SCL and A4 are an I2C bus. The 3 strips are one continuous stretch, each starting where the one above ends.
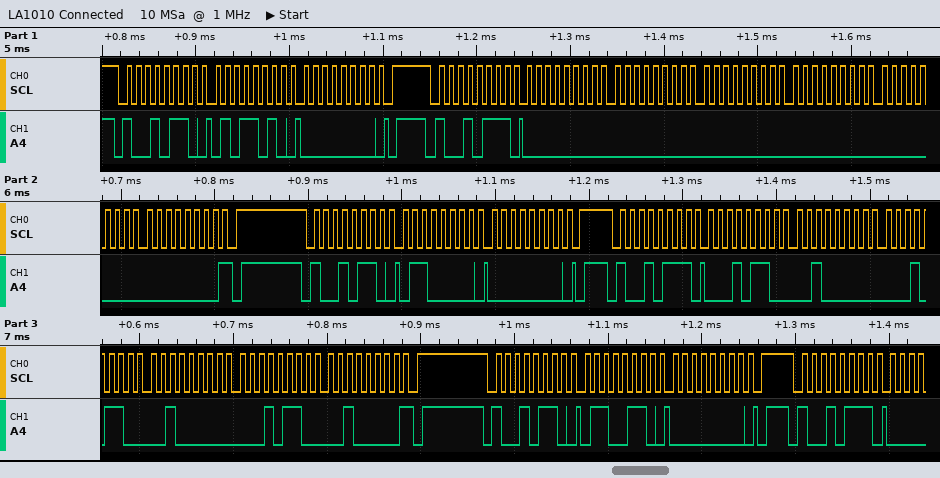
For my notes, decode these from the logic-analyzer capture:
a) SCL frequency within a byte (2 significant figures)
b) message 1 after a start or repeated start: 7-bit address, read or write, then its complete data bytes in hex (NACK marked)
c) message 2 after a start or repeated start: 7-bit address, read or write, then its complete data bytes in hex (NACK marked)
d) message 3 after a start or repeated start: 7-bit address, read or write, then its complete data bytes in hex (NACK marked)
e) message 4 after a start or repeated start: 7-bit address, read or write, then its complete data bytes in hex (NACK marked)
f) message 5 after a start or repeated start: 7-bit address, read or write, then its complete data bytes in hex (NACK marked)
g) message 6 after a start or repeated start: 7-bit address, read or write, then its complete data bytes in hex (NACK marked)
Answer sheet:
100 kHz
0x4B write: 5A 00
0x4B read: 00 00 00 00 00 00 NACK
0x4B write: 60 00
0x4B read: 16 20 16 20 16 20 NACK
0x4B write: 66 00
0x4B read
